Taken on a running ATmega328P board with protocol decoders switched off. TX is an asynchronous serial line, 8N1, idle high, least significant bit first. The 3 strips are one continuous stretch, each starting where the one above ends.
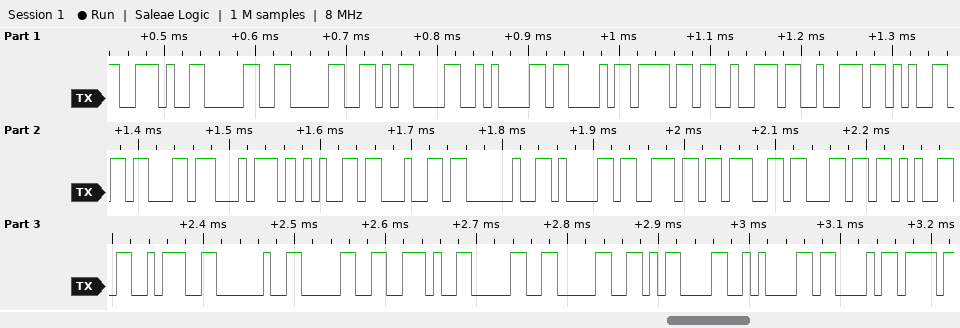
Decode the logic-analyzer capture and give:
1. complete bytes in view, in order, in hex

2E 30 30 0D 0A 43 6F 72 72 65 63 74 65 64 20 61 6E 67 6C 65 3A 20 30 2E 30 30 0D 0A 43
